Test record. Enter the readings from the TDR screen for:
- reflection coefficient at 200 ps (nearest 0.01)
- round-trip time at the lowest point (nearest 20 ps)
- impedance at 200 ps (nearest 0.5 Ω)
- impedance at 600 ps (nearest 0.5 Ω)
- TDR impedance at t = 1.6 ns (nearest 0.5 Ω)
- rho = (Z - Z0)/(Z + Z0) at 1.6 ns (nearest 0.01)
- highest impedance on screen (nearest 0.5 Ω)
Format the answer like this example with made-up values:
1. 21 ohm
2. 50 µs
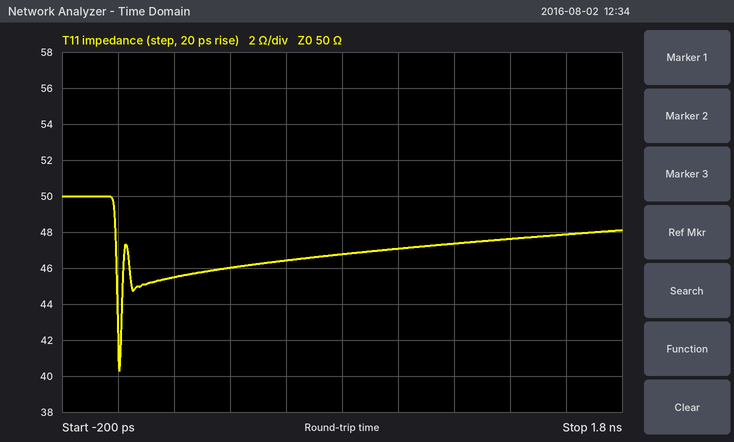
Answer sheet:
1. -0.05
2. 0 ps
3. 45.5 Ω
4. 46.5 Ω
5. 48.0 Ω
6. -0.02
7. 50.0 Ω
